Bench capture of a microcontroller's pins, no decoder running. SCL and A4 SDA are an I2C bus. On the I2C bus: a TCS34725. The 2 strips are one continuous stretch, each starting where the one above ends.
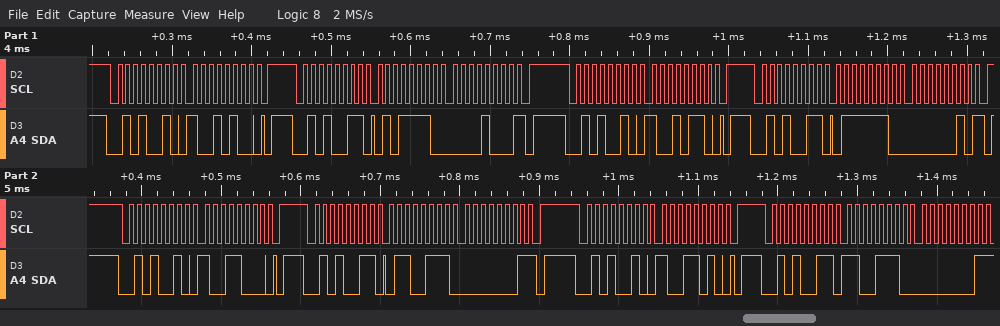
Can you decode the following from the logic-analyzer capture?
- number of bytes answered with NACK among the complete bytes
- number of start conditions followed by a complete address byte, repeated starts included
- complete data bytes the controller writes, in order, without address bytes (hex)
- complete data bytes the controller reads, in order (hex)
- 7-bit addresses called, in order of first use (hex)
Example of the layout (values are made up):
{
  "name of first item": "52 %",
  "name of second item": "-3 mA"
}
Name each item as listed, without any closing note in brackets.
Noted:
{
  "number of bytes answered with NACK among the complete bytes": "4",
  "number of start conditions followed by a complete address byte, repeated starts included": "8",
  "complete data bytes the controller writes, in order, without address bytes": "94 96 98 9A",
  "complete data bytes the controller reads, in order": "5E 08 7E 02 67 01 CE 01",
  "7-bit addresses called, in order of first use": "0x29"
}
